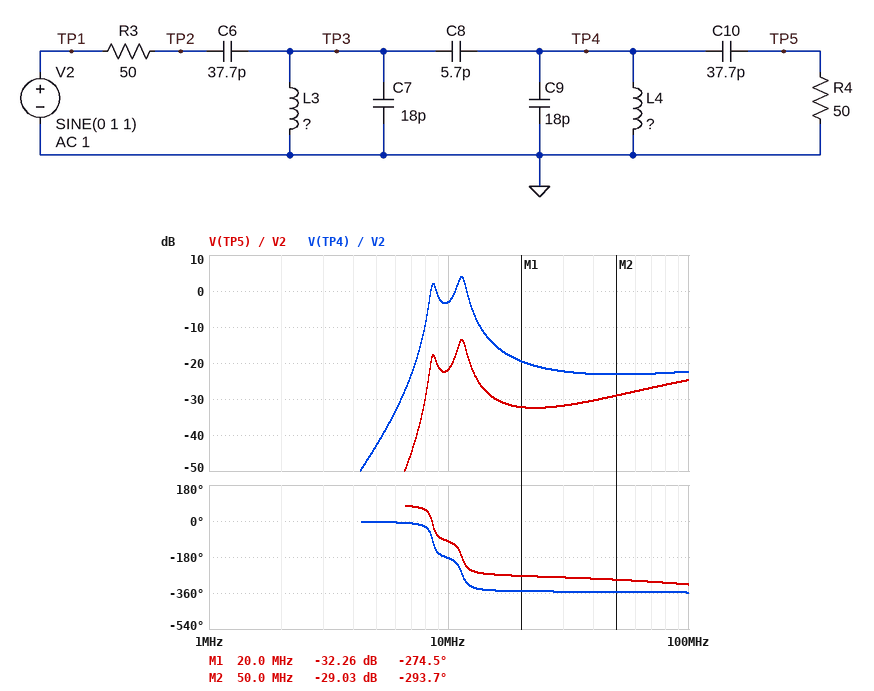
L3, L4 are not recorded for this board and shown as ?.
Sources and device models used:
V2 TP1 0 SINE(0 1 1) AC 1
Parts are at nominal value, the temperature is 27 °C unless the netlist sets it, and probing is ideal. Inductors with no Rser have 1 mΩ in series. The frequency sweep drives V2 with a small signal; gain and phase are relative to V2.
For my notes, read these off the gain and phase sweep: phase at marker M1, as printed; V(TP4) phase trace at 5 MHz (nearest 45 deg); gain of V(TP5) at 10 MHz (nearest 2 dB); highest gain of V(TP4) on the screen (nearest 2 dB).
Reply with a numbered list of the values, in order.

1. -274.5 deg
2. 0 deg
3. -22 dB
4. 4 dB
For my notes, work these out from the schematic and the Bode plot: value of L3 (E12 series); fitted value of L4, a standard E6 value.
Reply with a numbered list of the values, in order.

1. 5.6 µH
2. 3.3 µH
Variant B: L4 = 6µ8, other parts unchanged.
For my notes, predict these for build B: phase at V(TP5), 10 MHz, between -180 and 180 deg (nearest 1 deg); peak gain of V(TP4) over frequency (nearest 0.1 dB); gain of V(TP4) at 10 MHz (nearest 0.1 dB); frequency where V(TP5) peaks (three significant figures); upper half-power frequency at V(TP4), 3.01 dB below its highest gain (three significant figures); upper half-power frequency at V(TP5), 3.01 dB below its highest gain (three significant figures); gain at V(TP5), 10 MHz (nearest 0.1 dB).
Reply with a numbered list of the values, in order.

1. 105 deg
2. 11.1 dB
3. -4.6 dB
4. 8.73 MHz
5. 9.00 MHz
6. 9.01 MHz
7. -23.2 dB
